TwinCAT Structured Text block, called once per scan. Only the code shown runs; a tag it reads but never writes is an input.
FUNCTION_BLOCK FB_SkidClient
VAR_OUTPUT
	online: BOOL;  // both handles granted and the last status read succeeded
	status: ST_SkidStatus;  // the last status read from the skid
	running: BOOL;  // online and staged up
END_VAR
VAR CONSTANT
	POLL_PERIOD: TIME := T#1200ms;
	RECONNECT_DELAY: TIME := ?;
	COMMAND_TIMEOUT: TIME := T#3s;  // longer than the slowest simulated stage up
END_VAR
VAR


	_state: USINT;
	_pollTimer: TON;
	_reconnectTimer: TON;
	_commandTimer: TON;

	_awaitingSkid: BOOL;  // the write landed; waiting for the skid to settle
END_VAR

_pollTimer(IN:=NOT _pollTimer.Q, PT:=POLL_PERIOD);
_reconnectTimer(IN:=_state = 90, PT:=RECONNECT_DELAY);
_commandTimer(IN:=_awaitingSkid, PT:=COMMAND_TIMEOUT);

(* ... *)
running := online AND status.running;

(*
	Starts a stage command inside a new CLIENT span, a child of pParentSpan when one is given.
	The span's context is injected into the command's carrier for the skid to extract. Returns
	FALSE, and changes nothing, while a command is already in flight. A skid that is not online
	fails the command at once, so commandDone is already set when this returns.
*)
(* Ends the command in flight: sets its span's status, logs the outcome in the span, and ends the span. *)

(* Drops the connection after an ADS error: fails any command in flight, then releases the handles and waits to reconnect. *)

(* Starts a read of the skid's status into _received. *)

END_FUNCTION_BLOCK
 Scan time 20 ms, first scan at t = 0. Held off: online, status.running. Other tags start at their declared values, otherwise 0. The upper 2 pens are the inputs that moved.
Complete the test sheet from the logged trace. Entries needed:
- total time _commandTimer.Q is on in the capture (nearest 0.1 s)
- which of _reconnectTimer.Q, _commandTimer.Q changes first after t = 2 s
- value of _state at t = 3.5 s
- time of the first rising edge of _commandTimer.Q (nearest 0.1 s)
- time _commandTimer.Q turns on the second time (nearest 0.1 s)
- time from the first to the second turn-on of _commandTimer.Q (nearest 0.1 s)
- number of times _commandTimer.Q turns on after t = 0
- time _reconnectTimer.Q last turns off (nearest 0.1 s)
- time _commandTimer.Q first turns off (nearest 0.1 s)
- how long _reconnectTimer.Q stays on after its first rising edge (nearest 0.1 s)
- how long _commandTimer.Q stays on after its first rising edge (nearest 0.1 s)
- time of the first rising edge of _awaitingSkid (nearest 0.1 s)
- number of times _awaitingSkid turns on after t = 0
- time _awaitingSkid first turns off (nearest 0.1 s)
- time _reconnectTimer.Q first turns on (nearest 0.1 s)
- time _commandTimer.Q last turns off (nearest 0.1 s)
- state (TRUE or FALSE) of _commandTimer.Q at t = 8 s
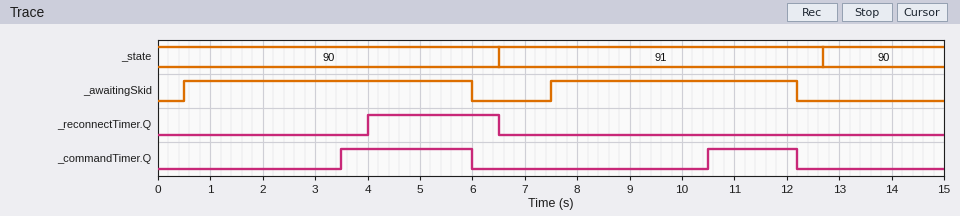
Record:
4.2 s
_commandTimer.Q
90
3.5 s
10.5 s
7.0 s
2
6.5 s
6.0 s
2.5 s
2.5 s
0.5 s
2
6.0 s
4.0 s
12.2 s
FALSE
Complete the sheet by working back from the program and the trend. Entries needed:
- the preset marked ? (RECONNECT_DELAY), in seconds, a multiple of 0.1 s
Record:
4.0 s
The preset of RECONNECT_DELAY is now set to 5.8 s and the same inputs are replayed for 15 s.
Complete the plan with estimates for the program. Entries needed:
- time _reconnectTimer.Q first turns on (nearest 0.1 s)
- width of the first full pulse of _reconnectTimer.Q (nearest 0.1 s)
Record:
5.8 s
0.7 s
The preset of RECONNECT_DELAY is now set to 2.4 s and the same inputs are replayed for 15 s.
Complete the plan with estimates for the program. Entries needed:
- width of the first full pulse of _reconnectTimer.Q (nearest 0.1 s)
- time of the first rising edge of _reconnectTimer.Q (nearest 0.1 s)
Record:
4.1 s
2.4 s
